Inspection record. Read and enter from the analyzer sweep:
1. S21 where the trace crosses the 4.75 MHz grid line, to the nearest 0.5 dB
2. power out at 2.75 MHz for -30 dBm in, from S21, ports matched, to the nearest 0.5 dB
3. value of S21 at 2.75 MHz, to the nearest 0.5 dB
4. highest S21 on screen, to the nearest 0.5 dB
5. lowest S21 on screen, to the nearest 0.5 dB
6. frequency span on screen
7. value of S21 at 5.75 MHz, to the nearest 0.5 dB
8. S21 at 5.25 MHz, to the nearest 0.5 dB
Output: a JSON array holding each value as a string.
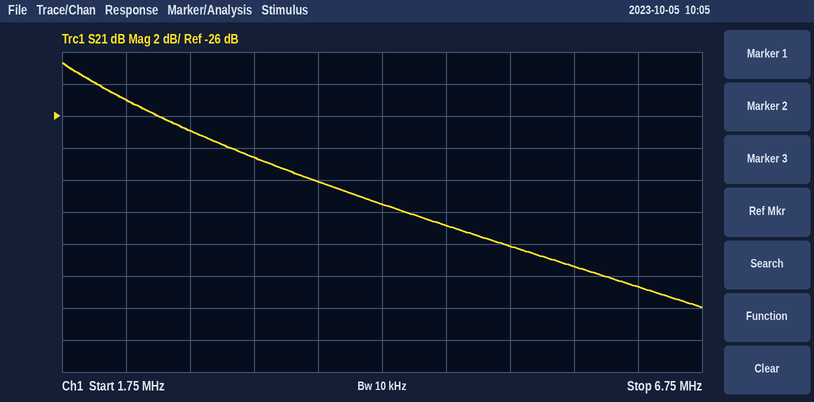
["-33.0 dB", "-57.0 dBm", "-27.0 dB", "-22.5 dB", "-38.0 dB", "5 MHz", "-35.5 dB", "-34.0 dB"]
